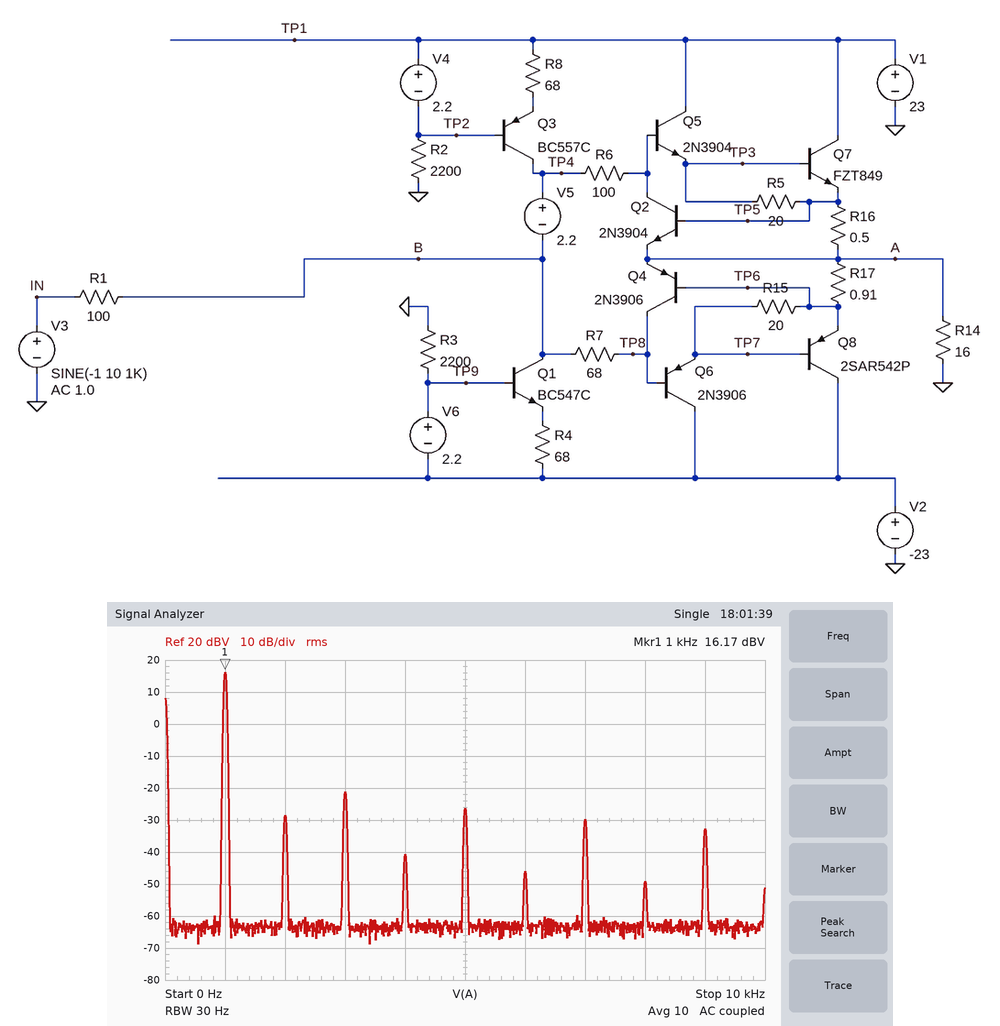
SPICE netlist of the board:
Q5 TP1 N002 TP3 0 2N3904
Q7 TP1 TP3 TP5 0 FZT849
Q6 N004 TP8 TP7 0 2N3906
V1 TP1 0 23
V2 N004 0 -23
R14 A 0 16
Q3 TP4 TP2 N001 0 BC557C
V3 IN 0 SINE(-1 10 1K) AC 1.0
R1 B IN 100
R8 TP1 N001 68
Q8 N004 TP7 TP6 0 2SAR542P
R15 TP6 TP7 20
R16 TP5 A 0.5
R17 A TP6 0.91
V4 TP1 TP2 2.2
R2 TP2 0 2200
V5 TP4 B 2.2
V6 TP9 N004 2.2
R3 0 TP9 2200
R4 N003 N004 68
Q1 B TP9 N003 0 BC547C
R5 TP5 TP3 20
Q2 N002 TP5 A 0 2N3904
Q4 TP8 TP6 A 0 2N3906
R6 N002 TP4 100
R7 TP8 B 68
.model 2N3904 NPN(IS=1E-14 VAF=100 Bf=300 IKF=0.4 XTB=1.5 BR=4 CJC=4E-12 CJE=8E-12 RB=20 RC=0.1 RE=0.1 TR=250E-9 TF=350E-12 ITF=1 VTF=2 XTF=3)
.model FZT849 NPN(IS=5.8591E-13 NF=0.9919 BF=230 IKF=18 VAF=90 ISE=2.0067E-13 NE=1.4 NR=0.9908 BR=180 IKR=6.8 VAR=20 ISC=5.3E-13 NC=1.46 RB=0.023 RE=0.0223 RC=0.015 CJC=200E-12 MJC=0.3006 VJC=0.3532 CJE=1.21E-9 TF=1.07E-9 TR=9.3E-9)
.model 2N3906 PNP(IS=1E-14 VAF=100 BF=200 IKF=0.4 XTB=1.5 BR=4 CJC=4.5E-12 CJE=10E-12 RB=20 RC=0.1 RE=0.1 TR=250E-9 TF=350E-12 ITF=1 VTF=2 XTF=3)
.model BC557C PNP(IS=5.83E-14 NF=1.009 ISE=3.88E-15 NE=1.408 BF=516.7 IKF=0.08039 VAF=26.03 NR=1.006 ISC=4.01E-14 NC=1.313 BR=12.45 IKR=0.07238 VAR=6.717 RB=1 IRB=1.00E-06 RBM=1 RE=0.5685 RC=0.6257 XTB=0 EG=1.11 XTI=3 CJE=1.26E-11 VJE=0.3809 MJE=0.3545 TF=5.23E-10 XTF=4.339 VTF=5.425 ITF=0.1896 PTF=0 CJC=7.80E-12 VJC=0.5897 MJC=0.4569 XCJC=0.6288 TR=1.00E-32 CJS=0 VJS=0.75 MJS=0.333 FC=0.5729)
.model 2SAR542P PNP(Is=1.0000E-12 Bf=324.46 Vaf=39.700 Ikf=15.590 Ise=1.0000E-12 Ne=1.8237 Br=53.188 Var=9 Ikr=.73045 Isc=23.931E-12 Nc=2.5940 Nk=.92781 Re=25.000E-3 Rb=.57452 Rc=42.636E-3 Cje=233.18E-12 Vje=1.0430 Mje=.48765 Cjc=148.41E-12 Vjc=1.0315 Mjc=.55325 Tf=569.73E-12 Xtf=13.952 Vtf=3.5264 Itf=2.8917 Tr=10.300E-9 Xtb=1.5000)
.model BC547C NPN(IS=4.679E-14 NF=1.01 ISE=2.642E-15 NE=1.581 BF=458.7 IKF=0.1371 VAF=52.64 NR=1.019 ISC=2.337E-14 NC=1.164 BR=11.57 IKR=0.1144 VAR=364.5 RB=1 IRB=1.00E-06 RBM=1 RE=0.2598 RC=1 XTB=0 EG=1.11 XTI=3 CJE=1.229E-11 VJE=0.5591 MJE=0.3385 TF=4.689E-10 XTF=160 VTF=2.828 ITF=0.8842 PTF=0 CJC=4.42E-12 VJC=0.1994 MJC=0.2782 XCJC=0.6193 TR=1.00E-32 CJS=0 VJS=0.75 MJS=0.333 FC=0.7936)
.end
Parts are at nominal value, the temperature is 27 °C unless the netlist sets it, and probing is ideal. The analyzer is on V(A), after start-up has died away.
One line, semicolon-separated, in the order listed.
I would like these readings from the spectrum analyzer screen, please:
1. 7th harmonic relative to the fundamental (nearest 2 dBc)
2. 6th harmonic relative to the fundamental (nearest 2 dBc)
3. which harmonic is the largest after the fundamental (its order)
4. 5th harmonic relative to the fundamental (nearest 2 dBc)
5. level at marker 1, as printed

-46 dBc; -62 dBc; 3; -42 dBc; 16.17 dBV
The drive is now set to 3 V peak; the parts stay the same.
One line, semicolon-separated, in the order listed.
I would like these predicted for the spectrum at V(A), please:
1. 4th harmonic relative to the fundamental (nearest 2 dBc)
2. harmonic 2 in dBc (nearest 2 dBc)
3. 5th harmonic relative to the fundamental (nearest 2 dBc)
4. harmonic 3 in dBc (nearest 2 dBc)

-48 dBc; -40 dBc; -36 dBc; -28 dBc
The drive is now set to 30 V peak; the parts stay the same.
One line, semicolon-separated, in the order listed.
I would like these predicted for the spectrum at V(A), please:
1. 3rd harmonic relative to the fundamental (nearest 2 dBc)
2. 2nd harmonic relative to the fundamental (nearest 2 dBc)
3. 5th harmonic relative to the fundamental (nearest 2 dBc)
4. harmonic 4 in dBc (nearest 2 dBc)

-16 dBc; -24 dBc; -48 dBc; -30 dBc
